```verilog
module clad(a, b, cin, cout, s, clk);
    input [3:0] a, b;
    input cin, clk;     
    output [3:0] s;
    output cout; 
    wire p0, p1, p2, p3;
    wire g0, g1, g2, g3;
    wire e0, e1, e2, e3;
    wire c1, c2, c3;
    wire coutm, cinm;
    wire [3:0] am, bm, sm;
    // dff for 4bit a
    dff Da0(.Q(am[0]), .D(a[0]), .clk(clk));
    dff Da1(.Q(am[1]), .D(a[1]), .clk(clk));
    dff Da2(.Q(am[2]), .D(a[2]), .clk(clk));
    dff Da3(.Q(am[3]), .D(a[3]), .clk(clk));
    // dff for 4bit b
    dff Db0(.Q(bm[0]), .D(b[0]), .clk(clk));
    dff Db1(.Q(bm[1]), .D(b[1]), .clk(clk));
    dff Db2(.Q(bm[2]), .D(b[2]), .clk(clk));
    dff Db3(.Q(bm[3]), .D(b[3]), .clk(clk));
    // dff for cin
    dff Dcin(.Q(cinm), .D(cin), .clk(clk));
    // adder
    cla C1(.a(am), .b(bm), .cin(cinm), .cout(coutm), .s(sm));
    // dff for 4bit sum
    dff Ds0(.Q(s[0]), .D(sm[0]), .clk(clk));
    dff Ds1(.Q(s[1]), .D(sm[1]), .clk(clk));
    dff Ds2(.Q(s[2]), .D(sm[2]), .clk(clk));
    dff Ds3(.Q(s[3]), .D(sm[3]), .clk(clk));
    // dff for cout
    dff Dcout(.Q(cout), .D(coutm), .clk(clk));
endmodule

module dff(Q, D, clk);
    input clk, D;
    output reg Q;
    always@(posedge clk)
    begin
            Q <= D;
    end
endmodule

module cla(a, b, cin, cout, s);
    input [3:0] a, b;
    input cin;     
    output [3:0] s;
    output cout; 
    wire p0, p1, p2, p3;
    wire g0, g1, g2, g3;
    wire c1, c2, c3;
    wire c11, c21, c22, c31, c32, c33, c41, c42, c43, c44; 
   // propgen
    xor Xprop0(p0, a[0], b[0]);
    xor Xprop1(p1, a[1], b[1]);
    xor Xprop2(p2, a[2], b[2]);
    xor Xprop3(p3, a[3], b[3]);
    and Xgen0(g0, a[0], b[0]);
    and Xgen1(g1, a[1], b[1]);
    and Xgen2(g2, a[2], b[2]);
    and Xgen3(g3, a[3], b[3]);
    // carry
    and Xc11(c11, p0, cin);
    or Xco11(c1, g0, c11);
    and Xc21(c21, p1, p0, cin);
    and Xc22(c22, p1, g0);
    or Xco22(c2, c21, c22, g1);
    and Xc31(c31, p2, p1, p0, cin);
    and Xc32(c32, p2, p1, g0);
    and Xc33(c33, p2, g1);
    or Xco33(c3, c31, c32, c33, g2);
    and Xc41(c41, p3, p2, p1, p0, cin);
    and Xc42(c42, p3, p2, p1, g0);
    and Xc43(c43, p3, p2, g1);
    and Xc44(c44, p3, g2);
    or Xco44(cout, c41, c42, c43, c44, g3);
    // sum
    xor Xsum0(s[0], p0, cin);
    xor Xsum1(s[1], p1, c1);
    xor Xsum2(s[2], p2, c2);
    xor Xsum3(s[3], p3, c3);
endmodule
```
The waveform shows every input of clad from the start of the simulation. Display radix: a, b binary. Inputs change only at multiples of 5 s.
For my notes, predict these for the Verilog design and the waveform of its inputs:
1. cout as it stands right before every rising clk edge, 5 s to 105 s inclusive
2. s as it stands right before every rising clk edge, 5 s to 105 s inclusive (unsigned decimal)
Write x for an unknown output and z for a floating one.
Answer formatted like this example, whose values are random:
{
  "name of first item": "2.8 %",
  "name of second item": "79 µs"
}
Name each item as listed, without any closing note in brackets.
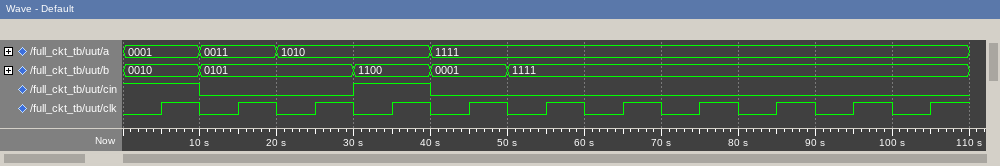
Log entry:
{
  "cout as it stands right before every rising clk edge, 5 s to 105 s inclusive": "x x 0 0 0 1 1 1 1 1 1",
  "s as it stands right before every rising clk edge, 5 s to 105 s inclusive": "x, x, 4, 8, 15, 7, 0, 14, 14, 14, 14"
}
